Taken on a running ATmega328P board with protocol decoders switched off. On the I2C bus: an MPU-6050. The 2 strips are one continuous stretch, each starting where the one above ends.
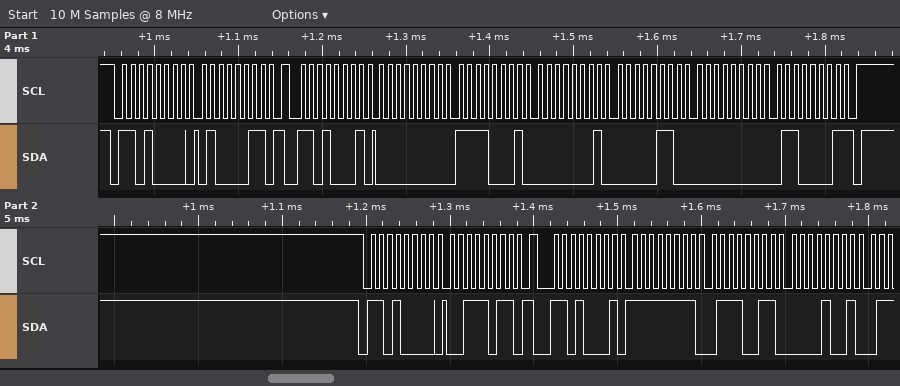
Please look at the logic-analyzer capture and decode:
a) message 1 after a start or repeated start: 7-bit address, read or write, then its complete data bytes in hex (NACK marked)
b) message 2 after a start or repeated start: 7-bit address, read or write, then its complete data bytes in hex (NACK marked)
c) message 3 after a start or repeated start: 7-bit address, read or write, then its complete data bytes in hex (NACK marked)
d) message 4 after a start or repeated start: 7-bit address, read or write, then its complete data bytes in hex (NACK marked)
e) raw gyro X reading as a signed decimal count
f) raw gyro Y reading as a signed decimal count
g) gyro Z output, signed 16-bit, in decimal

0x68 write: 43
0x68 read: 00 F1 01 06 00 61 NACK
0x68 write: 3B
0x68 read: FF 73 09
241
262
97
